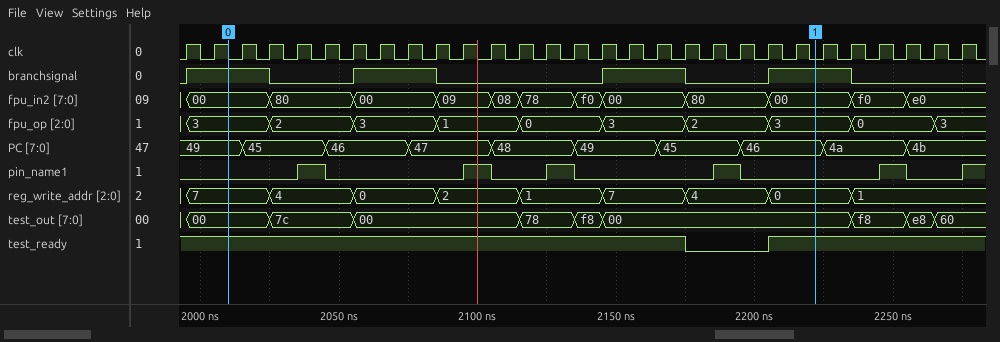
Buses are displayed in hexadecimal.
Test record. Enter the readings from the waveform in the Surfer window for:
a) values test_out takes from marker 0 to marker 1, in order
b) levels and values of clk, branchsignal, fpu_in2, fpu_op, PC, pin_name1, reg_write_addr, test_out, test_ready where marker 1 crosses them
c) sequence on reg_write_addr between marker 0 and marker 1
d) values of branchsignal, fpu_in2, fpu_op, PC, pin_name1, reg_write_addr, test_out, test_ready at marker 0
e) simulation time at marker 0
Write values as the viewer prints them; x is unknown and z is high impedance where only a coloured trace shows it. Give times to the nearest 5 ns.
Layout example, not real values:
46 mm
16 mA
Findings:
00, 7c, 00, 78, f8, 00
clk=0, branchsignal=1, fpu_in2=00, fpu_op=3, PC=46, pin_name1=0, reg_write_addr=0, test_out=00, test_ready=1
7, 4, 0, 2, 1, 7, 4, 0
branchsignal=1, fpu_in2=00, fpu_op=3, PC=49, pin_name1=0, reg_write_addr=7, test_out=00, test_ready=1
2010 ns
